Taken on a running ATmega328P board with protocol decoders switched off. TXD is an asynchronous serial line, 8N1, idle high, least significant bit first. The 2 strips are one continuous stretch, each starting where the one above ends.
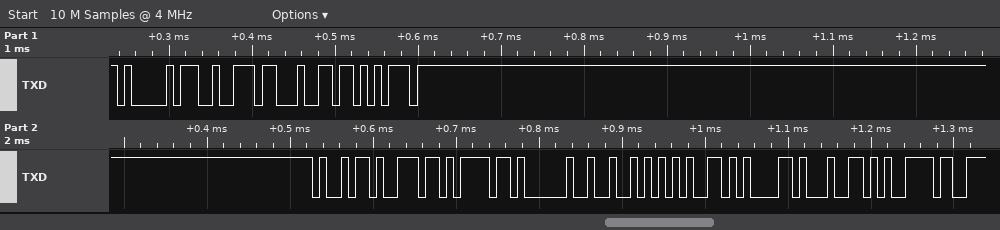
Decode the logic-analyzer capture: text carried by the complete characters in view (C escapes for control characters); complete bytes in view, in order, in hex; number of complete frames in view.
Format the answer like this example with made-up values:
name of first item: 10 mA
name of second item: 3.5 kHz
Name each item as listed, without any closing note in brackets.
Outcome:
text carried by the complete characters in view: "Arduino Ready"
complete bytes in view, in order, in hex: 41 72 64 75 69 6E 6F 20 52 65 61 64 79
number of complete frames in view: 13
